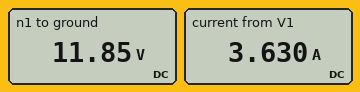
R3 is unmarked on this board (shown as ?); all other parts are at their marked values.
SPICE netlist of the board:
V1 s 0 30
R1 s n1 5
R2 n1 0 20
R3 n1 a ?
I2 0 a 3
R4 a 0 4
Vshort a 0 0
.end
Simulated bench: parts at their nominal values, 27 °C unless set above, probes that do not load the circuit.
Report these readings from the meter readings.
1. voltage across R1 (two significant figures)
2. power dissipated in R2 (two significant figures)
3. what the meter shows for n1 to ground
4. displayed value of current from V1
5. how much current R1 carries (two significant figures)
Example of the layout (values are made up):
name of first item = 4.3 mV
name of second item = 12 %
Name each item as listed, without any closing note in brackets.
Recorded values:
voltage across R1 = 18 V
power dissipated in R2 = 7.0 W
what the meter shows for n1 to ground = 11.85 V
displayed value of current from V1 = 3.630 A
how much current R1 carries = 3.6 A
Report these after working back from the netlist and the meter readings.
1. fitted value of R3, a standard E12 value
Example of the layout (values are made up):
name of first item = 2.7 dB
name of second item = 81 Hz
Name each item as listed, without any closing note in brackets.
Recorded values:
fitted value of R3, a standard E12 value = 3.9 Ω
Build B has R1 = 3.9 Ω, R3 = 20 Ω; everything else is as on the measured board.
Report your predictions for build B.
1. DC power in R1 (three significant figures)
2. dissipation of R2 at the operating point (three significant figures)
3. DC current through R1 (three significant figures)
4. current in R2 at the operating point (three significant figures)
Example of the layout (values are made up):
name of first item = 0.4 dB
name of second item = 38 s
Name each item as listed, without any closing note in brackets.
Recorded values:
DC power in R1 = 18.2 W
dissipation of R2 at the operating point = 23.3 W
DC current through R1 = 2.16 A
current in R2 at the operating point = 1.08 A
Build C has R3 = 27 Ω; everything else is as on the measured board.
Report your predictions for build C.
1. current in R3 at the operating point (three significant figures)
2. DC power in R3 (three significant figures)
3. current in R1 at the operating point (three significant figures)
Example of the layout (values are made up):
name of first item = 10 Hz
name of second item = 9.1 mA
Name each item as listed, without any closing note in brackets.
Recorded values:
current in R3 at the operating point = 774 mA
DC power in R3 = 16.2 W
current in R1 at the operating point = 1.82 A
